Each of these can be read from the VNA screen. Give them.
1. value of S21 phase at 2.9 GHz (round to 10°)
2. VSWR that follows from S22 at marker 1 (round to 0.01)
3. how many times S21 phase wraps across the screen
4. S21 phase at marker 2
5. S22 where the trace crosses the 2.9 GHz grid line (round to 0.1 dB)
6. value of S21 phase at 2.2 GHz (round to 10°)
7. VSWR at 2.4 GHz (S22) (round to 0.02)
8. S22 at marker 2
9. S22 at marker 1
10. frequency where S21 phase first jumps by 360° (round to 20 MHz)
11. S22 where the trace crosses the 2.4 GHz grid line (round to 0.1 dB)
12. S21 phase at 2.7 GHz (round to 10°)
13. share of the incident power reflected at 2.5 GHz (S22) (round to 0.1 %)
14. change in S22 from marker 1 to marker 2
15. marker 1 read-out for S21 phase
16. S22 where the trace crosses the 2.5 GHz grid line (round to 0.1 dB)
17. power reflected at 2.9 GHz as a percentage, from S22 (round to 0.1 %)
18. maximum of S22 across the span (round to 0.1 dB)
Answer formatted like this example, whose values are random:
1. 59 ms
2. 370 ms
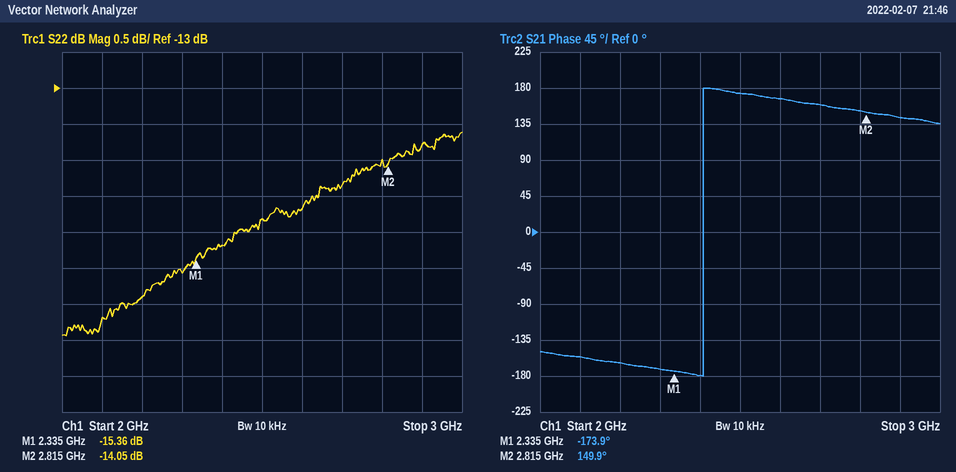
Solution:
1. 140°
2. 1.41
3. 1
4. 149.9°
5. -13.8 dB
6. -160°
7. 1.42
8. -14.05 dB
9. -15.36 dB
10. 2.40 GHz
11. -15.2 dB
12. 160°
13. 3.3 %
14. 1.31 dB
15. -173.9°
16. -14.8 dB
17. 4.2 %
18. -13.6 dB
